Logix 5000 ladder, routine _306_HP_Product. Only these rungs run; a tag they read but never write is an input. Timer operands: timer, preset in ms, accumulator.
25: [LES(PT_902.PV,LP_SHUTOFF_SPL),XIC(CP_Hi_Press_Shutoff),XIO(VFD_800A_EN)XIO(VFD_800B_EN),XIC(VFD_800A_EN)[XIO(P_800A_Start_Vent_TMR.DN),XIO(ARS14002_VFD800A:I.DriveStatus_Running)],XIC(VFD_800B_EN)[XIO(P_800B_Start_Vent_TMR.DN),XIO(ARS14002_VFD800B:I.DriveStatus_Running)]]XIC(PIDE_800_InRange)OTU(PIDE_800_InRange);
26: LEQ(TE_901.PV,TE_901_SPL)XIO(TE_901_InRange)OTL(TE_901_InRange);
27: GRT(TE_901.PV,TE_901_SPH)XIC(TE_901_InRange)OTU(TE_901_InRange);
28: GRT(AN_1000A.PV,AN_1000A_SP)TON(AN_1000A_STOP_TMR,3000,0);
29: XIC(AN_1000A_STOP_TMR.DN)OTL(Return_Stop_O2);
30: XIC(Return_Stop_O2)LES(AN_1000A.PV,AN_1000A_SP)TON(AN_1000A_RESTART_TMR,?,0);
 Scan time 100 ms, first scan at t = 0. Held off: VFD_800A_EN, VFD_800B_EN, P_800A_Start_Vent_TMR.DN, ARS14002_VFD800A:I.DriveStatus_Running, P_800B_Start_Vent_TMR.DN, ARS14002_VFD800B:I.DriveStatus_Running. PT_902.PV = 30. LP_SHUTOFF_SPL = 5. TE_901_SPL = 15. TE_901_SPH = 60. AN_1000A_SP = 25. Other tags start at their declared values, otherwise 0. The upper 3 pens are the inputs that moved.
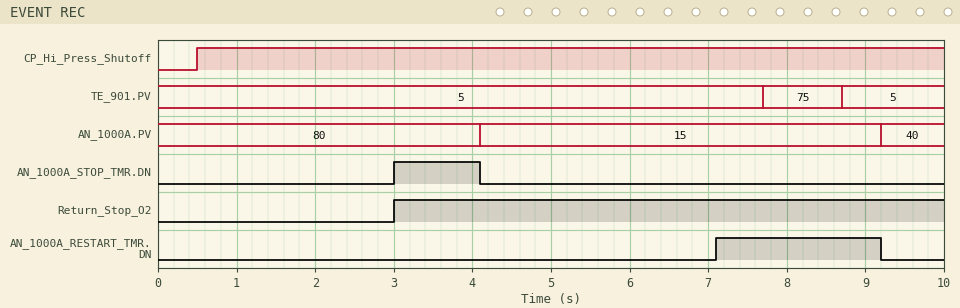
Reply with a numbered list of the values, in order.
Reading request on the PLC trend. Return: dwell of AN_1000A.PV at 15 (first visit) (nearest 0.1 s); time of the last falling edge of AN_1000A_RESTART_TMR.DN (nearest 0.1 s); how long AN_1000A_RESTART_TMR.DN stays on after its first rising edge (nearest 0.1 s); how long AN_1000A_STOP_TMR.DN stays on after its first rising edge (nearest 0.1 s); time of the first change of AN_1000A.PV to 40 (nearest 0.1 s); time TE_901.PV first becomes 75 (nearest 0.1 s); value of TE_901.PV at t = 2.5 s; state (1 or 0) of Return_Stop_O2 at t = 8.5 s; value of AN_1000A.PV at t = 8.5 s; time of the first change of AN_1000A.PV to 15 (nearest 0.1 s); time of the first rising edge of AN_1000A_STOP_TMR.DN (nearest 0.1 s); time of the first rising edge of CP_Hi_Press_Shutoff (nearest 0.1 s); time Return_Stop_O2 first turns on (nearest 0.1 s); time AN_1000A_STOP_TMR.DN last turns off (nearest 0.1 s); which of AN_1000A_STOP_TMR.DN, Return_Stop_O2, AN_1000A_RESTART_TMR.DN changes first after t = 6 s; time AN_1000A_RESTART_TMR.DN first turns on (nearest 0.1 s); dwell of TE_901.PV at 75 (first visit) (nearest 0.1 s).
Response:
1. 5.1 s
2. 9.2 s
3. 2.1 s
4. 1.1 s
5. 9.2 s
6. 7.7 s
7. 5
8. 1
9. 15
10. 4.1 s
11. 3.0 s
12. 0.5 s
13. 3.0 s
14. 4.1 s
15. AN_1000A_RESTART_TMR.DN
16. 7.1 s
17. 1.0 s
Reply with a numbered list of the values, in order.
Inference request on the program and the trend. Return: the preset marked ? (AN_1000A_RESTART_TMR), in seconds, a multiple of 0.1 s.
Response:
1. 3.0 s
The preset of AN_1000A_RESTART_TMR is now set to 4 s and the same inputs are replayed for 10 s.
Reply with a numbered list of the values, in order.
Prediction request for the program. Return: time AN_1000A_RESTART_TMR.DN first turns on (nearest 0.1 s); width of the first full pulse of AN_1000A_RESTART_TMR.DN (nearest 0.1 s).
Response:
1. 8.1 s
2. 1.1 s
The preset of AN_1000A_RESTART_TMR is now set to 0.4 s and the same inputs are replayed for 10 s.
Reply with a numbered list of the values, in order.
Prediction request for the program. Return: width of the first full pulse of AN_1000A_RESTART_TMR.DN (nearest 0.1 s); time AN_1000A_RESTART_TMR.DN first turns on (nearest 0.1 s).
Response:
1. 4.7 s
2. 4.5 s
